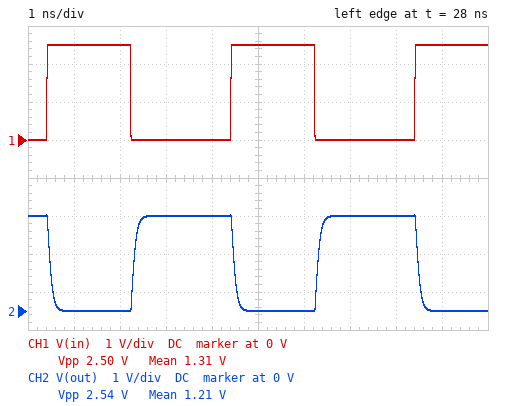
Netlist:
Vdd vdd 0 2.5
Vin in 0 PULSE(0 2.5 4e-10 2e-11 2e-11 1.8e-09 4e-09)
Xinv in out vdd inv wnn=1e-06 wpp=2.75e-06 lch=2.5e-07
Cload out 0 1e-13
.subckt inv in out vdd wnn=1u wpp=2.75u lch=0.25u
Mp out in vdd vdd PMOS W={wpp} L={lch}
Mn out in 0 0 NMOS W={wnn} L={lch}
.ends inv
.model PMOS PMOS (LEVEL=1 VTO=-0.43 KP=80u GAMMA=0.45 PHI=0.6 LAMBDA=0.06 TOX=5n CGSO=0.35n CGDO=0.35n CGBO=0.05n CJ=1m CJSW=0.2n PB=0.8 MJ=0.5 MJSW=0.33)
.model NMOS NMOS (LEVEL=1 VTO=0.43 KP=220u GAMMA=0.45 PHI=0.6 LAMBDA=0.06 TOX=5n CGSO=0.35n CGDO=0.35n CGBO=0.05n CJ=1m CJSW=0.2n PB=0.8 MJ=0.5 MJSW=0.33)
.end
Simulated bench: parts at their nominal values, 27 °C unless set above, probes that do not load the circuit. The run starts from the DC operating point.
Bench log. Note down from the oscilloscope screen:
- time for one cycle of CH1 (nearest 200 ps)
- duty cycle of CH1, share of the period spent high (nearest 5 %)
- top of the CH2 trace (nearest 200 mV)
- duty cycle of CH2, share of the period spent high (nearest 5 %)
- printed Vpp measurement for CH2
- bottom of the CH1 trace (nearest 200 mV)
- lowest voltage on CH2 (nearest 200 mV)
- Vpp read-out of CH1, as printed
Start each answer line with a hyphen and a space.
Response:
- 4.0 ns
- 45 %
- 2.6 V
- 55 %
- 2.54 V
- 0 V
- 0 V
- 2.50 V
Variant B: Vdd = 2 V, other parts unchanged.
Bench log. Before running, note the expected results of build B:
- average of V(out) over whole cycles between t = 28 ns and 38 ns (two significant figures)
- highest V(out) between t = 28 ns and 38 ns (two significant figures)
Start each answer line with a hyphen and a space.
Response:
- 1.1 V
- 2.0 V
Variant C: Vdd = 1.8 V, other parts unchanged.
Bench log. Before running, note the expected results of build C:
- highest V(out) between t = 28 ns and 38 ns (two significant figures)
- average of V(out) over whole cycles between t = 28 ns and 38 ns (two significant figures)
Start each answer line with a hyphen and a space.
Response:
- 1.8 V
- 950 mV
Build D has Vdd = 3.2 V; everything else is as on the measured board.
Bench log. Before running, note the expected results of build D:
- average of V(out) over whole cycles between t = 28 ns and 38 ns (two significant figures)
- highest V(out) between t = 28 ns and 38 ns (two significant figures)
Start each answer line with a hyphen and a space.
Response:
- 1.8 V
- 3.2 V
